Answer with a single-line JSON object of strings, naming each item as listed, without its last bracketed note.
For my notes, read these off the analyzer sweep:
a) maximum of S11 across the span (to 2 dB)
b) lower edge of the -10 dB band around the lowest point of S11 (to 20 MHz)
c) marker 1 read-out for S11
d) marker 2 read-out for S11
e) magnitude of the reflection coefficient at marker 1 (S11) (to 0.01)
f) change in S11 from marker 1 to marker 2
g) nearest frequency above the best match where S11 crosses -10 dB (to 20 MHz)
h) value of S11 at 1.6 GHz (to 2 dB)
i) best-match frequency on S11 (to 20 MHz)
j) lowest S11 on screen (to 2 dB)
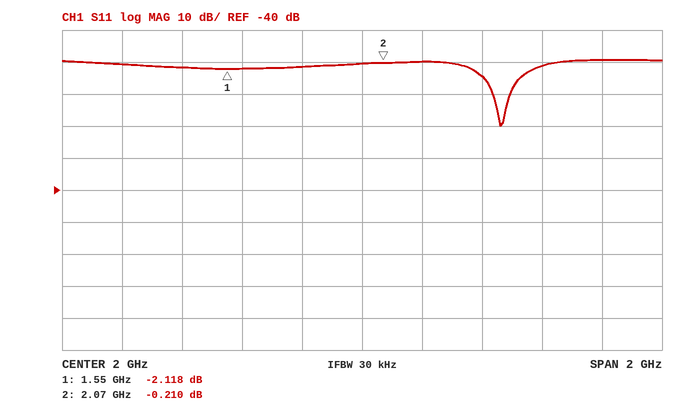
{"maximum of S11 across the span": "0 dB", "lower edge of the -10 dB band around the lowest point of S11": "2.44 GHz", "marker 1 read-out for S11": "-2.118 dB", "marker 2 read-out for S11": "-0.210 dB", "magnitude of the reflection coefficient at marker 1 (S11)": "0.78", "change in S11 from marker 1 to marker 2": "1.908 dB", "nearest frequency above the best match where S11 crosses -10 dB": "2.50 GHz", "value of S11 at 1.6 GHz": "-2 dB", "best-match frequency on S11": "2.46 GHz", "lowest S11 on screen": "-20 dB"}
